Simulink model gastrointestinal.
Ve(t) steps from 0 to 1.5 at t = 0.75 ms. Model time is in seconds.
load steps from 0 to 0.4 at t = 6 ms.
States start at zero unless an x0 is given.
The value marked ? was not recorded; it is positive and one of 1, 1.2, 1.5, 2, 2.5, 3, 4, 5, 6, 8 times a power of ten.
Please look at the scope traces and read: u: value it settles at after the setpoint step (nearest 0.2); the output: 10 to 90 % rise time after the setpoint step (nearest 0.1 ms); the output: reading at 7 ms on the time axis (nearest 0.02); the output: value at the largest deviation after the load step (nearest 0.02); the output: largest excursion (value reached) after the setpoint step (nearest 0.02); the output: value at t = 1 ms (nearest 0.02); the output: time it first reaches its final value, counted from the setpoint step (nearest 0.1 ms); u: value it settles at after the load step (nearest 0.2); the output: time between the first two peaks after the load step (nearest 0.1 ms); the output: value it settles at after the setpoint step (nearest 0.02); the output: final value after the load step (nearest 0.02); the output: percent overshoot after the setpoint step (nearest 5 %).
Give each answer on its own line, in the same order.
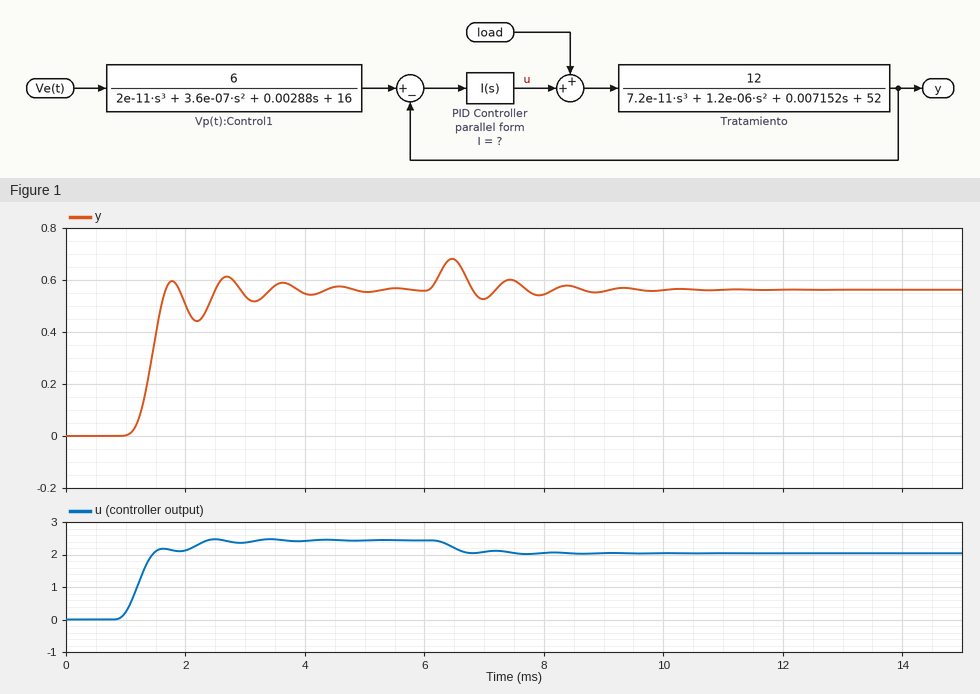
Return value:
2.4
0.4 ms
0.52
0.68
0.62
0.00
0.9 ms
2.0
1.0 ms
0.56
0.56
10 %
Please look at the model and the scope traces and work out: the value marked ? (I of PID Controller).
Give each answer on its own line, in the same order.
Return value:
8000
